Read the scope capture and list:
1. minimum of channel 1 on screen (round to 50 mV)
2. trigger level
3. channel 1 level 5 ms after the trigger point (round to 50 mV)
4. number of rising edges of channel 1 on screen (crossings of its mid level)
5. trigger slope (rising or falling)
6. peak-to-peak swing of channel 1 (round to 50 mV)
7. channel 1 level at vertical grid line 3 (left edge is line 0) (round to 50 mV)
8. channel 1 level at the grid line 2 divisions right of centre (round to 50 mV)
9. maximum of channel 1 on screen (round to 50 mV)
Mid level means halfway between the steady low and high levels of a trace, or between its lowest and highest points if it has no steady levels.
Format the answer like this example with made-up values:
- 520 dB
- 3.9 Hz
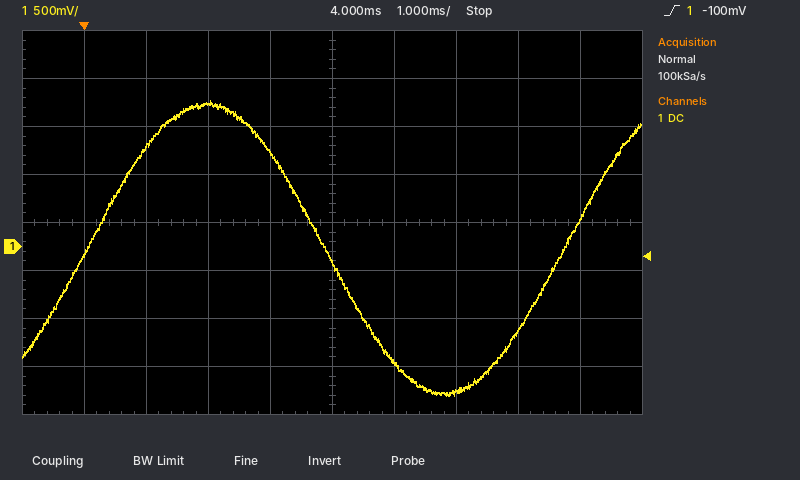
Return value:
- -1.55 V
- -100 mV
- -1.20 V
- 2
- rising
- 3.05 V
- 1.50 V
- -1.50 V
- 1.50 V
